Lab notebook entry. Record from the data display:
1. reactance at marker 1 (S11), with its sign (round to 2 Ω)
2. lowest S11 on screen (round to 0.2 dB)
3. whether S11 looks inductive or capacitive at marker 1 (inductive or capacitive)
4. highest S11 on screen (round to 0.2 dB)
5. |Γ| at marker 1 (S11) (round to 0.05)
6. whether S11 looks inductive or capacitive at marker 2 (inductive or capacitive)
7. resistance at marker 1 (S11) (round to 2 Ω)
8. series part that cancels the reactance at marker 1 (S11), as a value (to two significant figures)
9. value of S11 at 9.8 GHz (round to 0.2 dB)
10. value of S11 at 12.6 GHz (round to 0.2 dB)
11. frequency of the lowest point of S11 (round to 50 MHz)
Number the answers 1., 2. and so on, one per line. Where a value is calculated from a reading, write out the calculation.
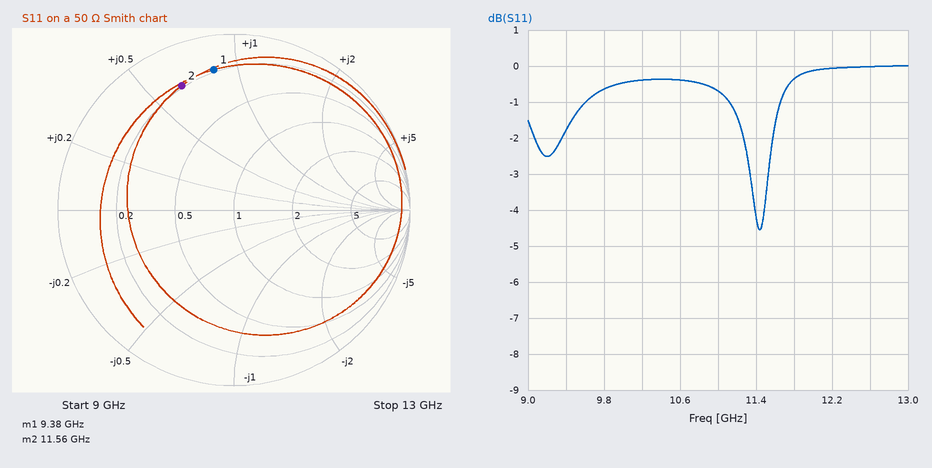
1. +42 Ω
2. -4.6 dB
3. inductive
4. 0.0 dB
5. 0.80
6. inductive
7. 10 Ω
8. C = 1/(2π × 9.38 GHz × 42 Ω) ≈ 404 fF, so 400 fF to two significant figures
9. -0.6 dB
10. 0.0 dB
11. 11.45 GHz
